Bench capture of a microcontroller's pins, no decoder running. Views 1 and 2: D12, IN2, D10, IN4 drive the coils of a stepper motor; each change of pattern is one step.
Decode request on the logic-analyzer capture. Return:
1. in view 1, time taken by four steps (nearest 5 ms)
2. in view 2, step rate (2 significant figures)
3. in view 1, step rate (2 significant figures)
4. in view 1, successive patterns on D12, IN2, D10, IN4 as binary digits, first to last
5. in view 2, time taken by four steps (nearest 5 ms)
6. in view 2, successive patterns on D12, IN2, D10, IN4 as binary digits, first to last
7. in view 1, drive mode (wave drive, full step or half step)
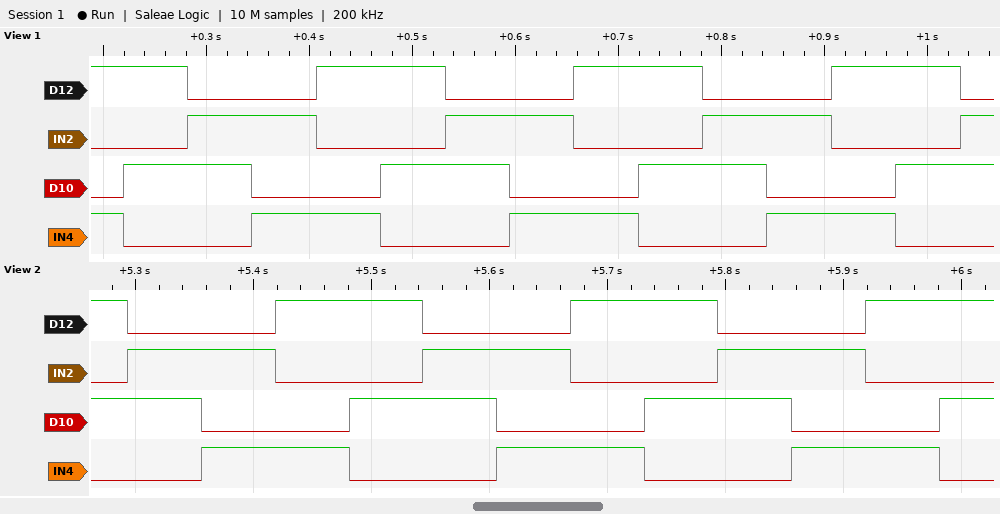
250 ms
16 steps/s
16 steps/s
1001 1010 0110 0101 1001 1010 0110 0101 1001 1010 0110 0101 1001 1010 0110
250 ms
1010 0110 0101 1001 1010 0110 0101 1001 1010 0110 0101 1001 1010
full step
